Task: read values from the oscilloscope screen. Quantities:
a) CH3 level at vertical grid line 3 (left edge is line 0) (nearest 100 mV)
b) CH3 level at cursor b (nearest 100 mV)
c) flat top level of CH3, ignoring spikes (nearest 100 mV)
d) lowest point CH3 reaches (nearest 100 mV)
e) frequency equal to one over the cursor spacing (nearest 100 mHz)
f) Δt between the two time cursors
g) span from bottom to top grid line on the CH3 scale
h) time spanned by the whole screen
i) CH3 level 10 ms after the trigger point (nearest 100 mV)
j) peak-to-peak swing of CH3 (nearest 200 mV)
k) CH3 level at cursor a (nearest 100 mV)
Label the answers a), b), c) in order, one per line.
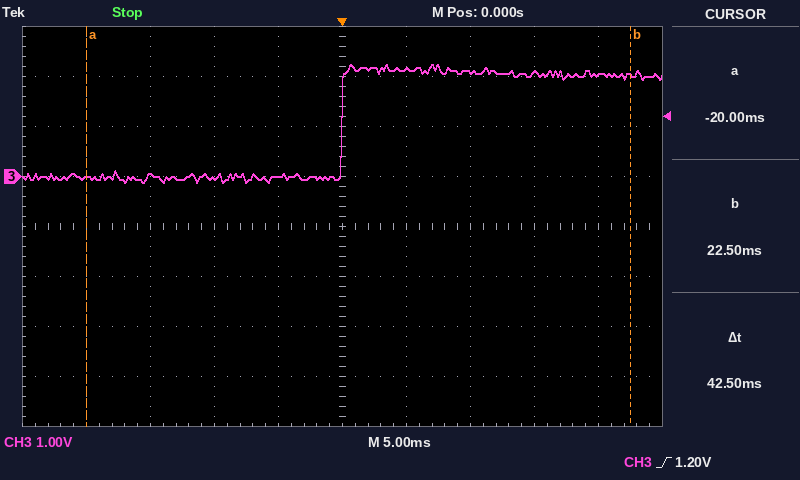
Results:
a) 0.0 V
b) 2.0 V
c) 2.1 V
d) -100 mV
e) 23.5 Hz
f) 42.5 ms
g) 8 V
h) 50 ms
i) 2.1 V
j) 2.4 V
k) 0.0 V
